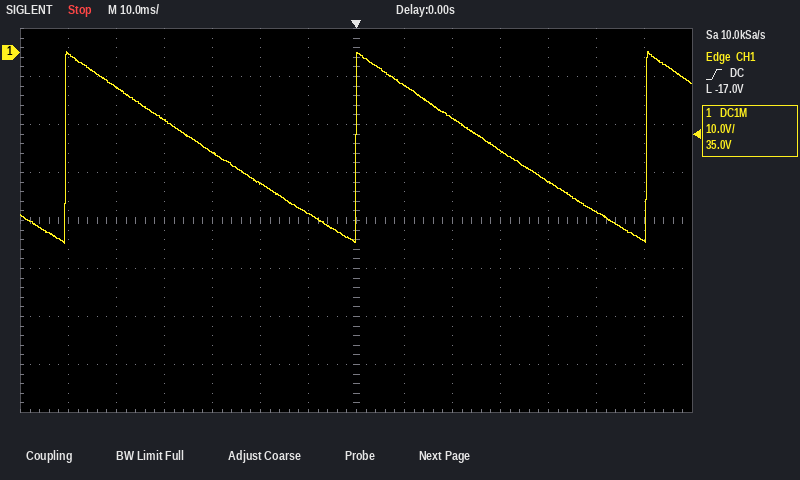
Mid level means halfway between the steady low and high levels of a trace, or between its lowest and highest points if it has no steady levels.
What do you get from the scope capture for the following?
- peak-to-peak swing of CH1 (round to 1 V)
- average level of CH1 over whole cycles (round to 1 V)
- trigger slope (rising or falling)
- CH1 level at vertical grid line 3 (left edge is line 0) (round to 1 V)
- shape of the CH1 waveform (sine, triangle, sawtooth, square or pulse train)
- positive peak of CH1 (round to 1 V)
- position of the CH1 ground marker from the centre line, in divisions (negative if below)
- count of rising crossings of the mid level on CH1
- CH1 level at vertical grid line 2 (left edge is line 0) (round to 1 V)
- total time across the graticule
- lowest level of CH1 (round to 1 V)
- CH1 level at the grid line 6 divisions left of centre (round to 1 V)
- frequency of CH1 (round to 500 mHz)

40 V
-20 V
rising
-14 V
sawtooth
0 V
+3.5 div
3
-7 V
140 ms
-40 V
0 V
16.5 Hz
